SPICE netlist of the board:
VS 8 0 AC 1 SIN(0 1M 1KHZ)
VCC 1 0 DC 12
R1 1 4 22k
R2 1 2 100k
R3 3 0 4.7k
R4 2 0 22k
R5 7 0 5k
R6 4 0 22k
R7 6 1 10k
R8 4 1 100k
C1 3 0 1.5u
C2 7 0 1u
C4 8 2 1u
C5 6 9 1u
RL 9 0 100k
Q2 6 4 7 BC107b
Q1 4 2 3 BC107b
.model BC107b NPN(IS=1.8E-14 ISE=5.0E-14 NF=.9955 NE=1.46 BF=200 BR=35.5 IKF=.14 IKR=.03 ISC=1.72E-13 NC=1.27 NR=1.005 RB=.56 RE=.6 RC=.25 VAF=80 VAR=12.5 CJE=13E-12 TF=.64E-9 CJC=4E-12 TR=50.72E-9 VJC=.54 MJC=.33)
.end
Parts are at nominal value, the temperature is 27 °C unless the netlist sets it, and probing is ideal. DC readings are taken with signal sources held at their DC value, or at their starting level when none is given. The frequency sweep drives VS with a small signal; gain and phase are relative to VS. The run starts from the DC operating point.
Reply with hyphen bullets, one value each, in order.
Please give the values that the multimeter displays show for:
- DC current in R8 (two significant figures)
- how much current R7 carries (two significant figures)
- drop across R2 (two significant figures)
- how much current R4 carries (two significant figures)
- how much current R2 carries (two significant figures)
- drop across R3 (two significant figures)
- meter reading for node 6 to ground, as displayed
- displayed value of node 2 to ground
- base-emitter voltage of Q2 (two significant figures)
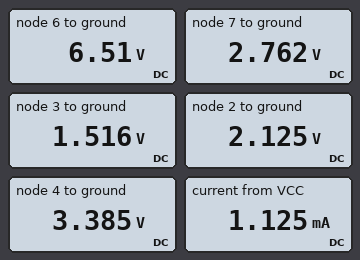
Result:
- 86 µA
- 550 µA
- 9.9 V
- 97 µA
- 99 µA
- 1.5 V
- 6.51 V
- 2.125 V
- 620 mV
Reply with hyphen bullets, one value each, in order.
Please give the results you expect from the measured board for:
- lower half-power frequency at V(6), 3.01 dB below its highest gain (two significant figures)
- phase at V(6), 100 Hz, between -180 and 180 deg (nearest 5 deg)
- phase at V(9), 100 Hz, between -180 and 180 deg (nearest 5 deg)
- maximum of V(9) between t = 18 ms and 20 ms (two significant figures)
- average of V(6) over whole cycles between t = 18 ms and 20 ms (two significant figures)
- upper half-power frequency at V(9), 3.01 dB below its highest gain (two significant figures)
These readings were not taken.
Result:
- 2.1 kHz
- 145 deg
- 145 deg
- 3.0 V
- 6.5 V
- 90 kHz
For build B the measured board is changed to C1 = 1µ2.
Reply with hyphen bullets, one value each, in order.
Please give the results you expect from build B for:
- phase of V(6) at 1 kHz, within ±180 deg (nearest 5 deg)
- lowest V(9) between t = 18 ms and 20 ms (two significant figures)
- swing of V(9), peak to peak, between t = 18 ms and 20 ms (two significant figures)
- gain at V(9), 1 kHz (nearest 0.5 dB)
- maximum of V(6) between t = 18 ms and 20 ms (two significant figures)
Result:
- 110 deg
- -2.9 V
- 5.5 V
- 69.0 dB
- 9.2 V
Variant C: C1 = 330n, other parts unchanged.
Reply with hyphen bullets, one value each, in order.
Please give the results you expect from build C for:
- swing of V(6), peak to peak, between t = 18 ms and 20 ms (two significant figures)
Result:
- 1.8 V
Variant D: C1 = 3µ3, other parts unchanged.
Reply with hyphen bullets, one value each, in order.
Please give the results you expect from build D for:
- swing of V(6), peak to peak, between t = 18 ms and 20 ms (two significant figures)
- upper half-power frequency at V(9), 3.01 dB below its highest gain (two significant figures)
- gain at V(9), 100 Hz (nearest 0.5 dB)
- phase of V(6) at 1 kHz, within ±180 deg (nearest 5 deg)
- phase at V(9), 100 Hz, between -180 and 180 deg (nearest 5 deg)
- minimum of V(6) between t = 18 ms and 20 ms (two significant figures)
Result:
- 7.6 V
- 89 kHz
- 41.0 dB
- 85 deg
- 150 deg
- 2.9 V
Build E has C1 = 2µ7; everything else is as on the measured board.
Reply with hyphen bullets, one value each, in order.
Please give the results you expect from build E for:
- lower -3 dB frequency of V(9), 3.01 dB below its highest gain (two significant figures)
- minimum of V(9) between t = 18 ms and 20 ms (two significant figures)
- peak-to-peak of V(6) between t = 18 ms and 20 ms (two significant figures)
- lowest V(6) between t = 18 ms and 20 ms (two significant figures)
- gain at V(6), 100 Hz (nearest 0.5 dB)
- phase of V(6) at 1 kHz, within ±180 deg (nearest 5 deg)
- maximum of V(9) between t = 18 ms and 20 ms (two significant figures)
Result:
- 1.7 kHz
- -3.6 V
- 7.4 V
- 2.9 V
- 39.5 dB
- 90 deg
- 3.8 V
